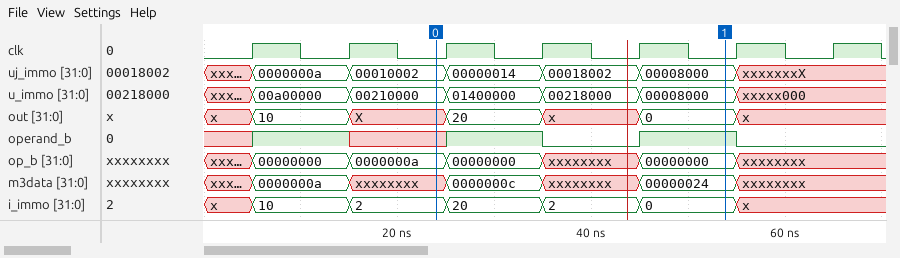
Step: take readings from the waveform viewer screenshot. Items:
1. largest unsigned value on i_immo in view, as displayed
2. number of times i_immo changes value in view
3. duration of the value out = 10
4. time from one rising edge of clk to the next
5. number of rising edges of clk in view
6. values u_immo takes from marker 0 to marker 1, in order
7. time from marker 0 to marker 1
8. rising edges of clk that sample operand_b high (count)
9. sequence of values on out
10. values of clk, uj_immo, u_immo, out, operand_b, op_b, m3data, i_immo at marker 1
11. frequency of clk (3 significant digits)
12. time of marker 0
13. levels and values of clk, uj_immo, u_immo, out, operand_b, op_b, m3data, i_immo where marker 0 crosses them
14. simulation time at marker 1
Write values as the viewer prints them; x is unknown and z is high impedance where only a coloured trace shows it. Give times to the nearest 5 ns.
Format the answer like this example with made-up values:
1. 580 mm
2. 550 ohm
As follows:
1. 20
2. 6
3. 10 ns
4. 10 ns
5. 7
6. 00210000, 01400000, 00218000, 00008000
7. 30 ns
8. 3
9. x, 10, X, 20, x, 0, x
10. clk=0, uj_immo=00008000, u_immo=00008000, out=0, operand_b=1, op_b=00000000, m3data=00000024, i_immo=0
11. 100 MHz
12. 25 ns
13. clk=0, uj_immo=00010002, u_immo=00210000, out=X, operand_b=x, op_b=0000000a, m3data=xxxxxxxx, i_immo=2
14. 55 ns
